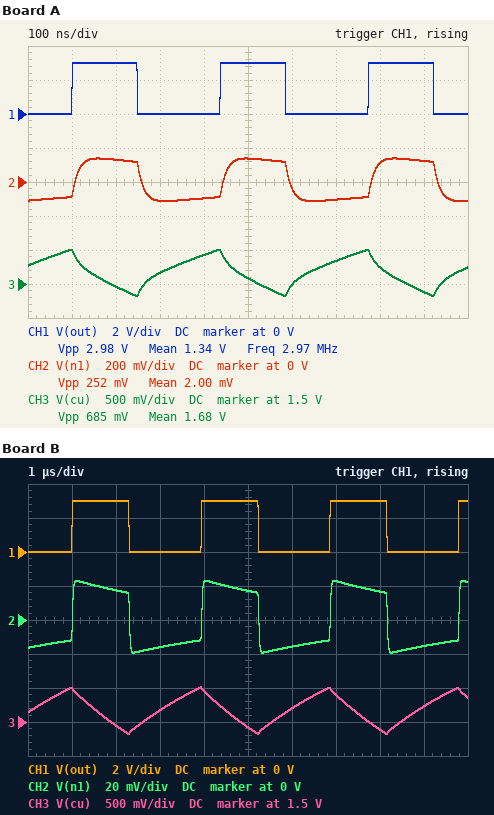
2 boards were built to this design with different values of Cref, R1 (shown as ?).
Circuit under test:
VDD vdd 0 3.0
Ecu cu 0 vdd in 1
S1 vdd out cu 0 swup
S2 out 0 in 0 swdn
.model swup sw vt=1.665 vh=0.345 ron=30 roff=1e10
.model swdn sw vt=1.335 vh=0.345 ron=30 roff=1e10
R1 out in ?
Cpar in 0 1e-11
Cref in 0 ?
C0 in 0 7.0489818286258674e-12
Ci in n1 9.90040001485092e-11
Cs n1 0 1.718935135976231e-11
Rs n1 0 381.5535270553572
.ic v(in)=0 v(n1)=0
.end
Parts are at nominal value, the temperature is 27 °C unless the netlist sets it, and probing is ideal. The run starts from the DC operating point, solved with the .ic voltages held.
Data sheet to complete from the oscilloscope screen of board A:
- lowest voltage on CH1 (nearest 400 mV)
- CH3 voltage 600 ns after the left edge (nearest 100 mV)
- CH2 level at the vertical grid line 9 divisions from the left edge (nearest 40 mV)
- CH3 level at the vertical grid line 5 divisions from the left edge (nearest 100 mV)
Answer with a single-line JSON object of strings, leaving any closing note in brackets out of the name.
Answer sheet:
{"lowest voltage on CH1": "0 V", "CH3 voltage 600 ns after the left edge": "1.5 V", "CH2 level at the vertical grid line 9 divisions from the left edge": "120 mV", "CH3 level at the vertical grid line 5 divisions from the left edge": "1.6 V"}
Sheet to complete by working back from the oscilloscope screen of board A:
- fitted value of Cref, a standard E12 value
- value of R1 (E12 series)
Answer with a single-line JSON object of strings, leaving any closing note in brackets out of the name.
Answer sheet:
{"fitted value of Cref, a standard E12 value": "15 pF", "value of R1": "3.3 kΩ"}
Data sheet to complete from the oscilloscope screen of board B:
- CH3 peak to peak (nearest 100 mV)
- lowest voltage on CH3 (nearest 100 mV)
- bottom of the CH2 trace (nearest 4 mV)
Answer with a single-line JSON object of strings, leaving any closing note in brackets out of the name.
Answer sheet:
{"CH3 peak to peak": "700 mV", "lowest voltage on CH3": "1.3 V", "bottom of the CH2 trace": "-20 mV"}
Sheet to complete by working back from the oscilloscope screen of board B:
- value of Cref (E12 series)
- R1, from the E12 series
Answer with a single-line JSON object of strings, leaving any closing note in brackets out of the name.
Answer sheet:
{"value of Cref": "27 pF", "R1, from the E12 series": "22 kΩ"}
